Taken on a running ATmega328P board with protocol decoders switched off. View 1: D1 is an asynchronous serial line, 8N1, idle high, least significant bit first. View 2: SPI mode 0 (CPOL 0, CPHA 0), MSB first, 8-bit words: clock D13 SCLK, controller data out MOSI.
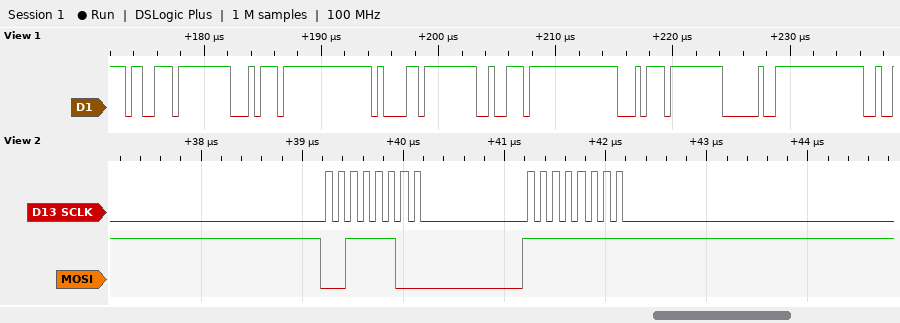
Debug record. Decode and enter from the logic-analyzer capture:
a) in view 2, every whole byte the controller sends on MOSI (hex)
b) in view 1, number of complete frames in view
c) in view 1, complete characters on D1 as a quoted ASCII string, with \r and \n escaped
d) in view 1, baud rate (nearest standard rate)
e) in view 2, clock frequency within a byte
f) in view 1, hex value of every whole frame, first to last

3C FF
6
"start "
2000000 baud
8 MHz
73 74 61 72 74 20
